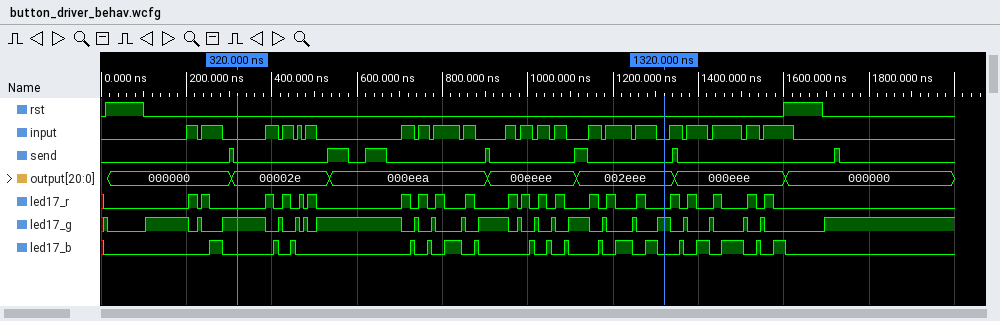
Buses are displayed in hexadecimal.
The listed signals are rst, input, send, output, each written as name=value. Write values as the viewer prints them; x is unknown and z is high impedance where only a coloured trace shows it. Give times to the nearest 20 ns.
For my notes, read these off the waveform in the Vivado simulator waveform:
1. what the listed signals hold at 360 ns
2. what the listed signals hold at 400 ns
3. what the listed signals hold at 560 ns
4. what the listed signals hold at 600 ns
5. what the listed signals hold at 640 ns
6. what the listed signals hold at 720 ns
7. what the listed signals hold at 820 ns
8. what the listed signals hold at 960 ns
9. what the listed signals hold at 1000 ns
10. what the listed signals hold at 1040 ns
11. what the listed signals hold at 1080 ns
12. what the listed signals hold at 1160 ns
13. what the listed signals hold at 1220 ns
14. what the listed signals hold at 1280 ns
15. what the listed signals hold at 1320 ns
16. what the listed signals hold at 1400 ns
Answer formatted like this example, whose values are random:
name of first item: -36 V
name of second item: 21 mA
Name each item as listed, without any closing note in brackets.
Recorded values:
what the listed signals hold at 360 ns: rst=0, input=0, send=0, output=00002e
what the listed signals hold at 400 ns: rst=0, input=1, send=0, output=00002e
what the listed signals hold at 560 ns: rst=0, input=0, send=1, output=000eea
what the listed signals hold at 600 ns: rst=0, input=0, send=0, output=000eea
what the listed signals hold at 640 ns: rst=0, input=0, send=1, output=000eea
what the listed signals hold at 720 ns: rst=0, input=1, send=0, output=000eea
what the listed signals hold at 820 ns: rst=0, input=1, send=0, output=000eea
what the listed signals hold at 960 ns: rst=0, input=1, send=0, output=00eeee
what the listed signals hold at 1000 ns: rst=0, input=1, send=0, output=00eeee
what the listed signals hold at 1040 ns: rst=0, input=1, send=0, output=00eeee
what the listed signals hold at 1080 ns: rst=0, input=1, send=0, output=00eeee
what the listed signals hold at 1160 ns: rst=0, input=1, send=0, output=002eee
what the listed signals hold at 1220 ns: rst=0, input=1, send=0, output=002eee
what the listed signals hold at 1280 ns: rst=0, input=1, send=0, output=002eee
what the listed signals hold at 1320 ns: rst=0, input=0, send=0, output=002eee
what the listed signals hold at 1400 ns: rst=0, input=1, send=0, output=000eee
